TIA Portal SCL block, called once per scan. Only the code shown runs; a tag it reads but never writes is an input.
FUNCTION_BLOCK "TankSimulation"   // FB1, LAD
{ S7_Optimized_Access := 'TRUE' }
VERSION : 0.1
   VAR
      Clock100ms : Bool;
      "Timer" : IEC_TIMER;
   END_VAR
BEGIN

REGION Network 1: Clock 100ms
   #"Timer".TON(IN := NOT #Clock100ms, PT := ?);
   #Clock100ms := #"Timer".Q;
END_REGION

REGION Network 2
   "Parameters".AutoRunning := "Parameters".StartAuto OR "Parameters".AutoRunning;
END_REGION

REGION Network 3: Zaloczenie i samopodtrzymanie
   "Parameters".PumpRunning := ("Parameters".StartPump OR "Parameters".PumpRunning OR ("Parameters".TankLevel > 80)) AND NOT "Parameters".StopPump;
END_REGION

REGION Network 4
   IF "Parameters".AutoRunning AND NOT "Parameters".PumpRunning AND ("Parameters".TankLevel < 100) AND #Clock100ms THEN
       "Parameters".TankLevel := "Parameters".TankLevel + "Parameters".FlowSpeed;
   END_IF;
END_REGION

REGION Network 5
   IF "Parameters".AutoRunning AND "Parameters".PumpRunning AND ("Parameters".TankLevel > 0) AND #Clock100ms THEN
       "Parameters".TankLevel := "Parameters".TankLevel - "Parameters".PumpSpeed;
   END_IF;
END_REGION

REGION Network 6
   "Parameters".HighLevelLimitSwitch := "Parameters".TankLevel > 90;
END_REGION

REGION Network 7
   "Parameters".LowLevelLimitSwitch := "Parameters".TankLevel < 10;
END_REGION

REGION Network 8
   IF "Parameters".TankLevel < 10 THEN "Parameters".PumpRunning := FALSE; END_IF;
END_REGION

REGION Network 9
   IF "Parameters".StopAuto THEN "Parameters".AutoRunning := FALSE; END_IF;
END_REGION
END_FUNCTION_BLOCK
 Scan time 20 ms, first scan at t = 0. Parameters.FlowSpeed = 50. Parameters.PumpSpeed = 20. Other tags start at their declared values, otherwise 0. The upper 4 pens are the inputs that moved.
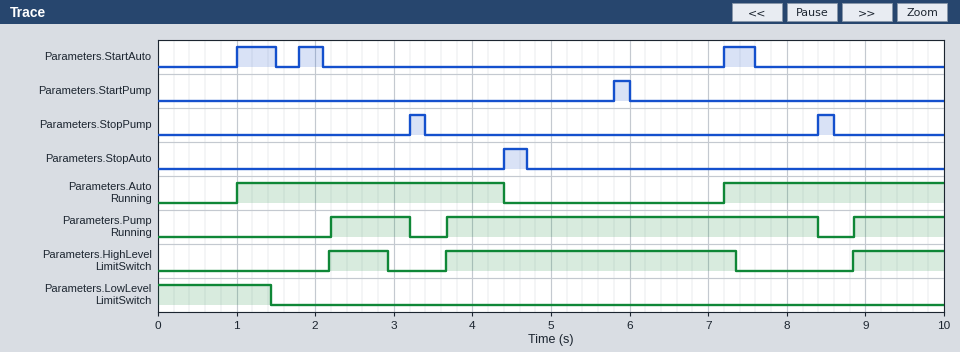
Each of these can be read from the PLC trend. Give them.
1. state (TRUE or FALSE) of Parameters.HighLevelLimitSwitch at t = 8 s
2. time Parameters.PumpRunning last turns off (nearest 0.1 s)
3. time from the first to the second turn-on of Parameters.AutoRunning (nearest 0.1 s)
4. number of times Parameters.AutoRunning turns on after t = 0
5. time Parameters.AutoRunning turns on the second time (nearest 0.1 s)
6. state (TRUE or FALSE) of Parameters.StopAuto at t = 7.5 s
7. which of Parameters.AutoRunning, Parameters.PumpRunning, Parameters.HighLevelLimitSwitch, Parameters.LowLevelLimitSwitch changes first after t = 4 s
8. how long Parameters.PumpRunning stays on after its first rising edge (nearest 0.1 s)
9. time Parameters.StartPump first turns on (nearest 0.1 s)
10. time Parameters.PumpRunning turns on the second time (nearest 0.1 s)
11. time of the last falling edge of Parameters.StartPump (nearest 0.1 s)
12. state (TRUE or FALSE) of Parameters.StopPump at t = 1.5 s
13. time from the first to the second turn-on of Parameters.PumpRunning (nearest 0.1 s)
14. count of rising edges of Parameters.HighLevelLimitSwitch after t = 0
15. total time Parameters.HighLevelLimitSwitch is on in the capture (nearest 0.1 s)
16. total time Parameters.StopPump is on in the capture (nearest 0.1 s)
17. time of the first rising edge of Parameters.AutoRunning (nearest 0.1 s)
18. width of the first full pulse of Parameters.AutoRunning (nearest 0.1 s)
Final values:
FALSE
8.4 s
6.2 s
2
7.2 s
FALSE
Parameters.AutoRunning
1.0 s
5.8 s
3.7 s
6.0 s
FALSE
1.5 s
3
5.6 s
0.4 s
1.0 s
3.4 s
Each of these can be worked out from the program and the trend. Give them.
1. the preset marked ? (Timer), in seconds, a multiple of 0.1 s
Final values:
0.7 s
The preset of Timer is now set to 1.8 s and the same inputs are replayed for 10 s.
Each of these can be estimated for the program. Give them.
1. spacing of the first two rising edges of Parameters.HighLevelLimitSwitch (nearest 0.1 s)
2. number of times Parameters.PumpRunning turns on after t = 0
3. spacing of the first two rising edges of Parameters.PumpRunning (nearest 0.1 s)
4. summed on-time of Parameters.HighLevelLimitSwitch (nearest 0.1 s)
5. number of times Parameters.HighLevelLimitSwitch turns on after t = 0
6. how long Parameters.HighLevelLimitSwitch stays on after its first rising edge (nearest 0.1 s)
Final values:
5.5 s
2
5.5 s
4.5 s
2
3.7 s
